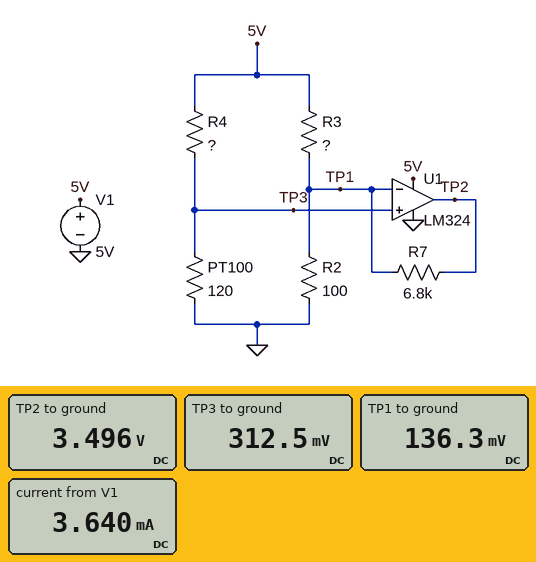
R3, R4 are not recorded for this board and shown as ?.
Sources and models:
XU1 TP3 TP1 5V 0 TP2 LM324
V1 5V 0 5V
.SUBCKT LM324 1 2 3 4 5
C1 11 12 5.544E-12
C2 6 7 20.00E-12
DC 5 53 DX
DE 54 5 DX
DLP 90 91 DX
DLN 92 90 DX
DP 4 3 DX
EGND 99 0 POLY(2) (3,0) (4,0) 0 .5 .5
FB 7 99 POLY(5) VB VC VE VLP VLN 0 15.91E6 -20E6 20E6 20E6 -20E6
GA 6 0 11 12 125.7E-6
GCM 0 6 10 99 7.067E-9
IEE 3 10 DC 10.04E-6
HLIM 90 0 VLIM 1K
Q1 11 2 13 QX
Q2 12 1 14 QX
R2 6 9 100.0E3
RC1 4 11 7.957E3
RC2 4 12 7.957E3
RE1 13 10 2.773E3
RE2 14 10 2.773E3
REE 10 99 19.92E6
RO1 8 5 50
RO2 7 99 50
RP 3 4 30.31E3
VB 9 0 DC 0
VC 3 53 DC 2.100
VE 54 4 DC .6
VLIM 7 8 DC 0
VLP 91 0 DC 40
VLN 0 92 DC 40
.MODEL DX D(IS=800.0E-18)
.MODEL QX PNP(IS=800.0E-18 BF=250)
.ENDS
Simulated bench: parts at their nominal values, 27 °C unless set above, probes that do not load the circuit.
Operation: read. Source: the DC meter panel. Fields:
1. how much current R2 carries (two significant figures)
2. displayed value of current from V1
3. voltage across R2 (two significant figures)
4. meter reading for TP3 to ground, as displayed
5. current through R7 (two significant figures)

1.4 mA
3.640 mA
140 mV
312.5 mV
490 µA
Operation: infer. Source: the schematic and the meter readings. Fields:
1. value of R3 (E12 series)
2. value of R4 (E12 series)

5.6 kΩ
1.8 kΩ
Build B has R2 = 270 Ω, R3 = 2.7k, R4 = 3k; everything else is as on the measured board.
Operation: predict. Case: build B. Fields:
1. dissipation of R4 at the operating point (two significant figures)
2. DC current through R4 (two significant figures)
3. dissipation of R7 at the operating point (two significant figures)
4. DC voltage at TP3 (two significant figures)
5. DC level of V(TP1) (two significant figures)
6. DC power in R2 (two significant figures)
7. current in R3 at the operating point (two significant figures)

7.7 mW
1.6 mA
28 µW
190 mV
440 mV
710 µW
1.7 mA
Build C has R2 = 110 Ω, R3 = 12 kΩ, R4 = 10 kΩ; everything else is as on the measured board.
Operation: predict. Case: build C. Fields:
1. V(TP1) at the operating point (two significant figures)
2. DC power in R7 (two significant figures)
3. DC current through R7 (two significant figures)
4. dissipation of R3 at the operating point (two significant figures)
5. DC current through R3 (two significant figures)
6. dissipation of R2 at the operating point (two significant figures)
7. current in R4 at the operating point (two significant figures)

59 mV
110 µW
130 µA
2.0 mW
410 µA
32 µW
490 µA
